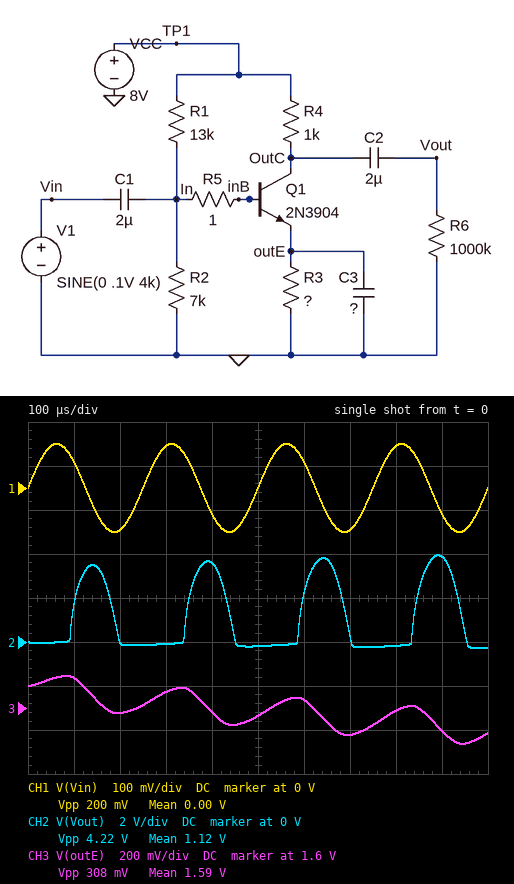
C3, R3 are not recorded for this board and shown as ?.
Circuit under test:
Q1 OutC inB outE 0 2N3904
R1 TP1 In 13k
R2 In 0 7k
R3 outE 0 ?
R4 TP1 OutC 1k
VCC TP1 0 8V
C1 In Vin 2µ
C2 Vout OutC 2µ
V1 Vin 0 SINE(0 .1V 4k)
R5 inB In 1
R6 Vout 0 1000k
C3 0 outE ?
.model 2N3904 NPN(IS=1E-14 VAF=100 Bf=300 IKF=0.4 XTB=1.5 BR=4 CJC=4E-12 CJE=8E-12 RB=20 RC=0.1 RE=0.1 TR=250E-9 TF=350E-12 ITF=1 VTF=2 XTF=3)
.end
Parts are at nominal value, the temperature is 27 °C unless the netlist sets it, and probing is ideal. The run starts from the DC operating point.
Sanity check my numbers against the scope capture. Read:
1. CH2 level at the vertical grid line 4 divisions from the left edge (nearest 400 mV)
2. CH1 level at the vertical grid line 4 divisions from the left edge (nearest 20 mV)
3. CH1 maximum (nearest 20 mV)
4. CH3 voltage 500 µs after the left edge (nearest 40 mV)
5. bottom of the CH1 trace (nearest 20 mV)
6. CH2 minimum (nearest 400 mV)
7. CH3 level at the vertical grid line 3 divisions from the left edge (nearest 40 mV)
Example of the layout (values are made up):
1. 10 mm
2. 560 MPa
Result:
1. 3.6 V
2. -60 mV
3. 100 mV
4. 1.56 V
5. -100 mV
6. -400 mV
7. 1.68 V
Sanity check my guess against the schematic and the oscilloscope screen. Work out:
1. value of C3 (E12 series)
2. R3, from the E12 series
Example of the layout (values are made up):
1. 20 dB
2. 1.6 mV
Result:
1. 1.5 µF
2. 270 Ω
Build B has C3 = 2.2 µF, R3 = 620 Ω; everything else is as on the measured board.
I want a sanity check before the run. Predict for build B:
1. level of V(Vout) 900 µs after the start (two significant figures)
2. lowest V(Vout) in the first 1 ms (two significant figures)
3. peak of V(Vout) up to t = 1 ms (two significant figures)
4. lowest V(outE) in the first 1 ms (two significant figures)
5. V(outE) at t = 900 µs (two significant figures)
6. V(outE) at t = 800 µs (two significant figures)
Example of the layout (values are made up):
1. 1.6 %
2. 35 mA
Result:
1. 3.1 V
2. -2.7 V
3. 3.2 V
4. 1.9 V
5. 2.0 V
6. 2.1 V
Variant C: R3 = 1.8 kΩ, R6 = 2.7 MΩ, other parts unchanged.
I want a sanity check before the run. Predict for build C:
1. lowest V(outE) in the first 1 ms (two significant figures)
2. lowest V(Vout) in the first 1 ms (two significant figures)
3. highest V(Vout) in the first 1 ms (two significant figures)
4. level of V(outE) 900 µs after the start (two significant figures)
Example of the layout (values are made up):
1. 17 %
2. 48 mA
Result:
1. 2.1 V
2. -3.1 V
3. 1.2 V
4. 2.2 V
